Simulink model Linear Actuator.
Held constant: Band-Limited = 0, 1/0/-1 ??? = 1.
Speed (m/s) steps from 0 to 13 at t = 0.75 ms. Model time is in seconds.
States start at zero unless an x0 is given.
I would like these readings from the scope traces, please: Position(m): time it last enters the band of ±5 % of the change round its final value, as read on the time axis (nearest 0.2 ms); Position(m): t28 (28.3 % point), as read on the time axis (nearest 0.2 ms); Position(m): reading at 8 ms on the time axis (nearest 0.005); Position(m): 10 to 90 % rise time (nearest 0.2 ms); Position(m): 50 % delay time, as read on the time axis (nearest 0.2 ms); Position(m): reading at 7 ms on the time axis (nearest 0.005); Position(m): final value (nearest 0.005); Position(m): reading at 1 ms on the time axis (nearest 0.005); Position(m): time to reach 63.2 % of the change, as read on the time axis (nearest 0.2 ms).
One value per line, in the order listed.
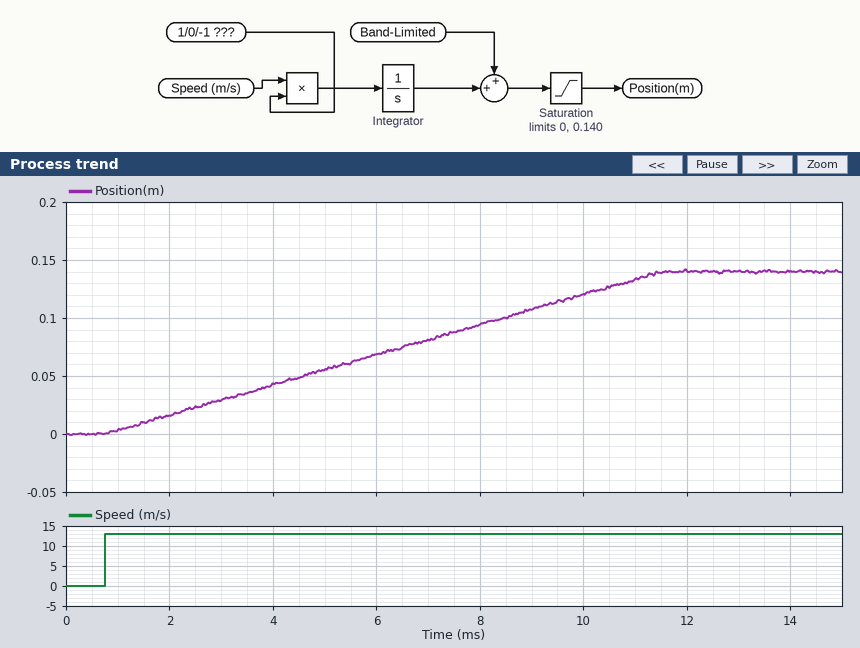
11.0 ms
3.8 ms
0.095
8.6 ms
6.2 ms
0.080
0.140
0.005
7.6 ms
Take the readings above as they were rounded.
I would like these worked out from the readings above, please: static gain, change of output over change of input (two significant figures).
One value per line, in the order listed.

0.011
